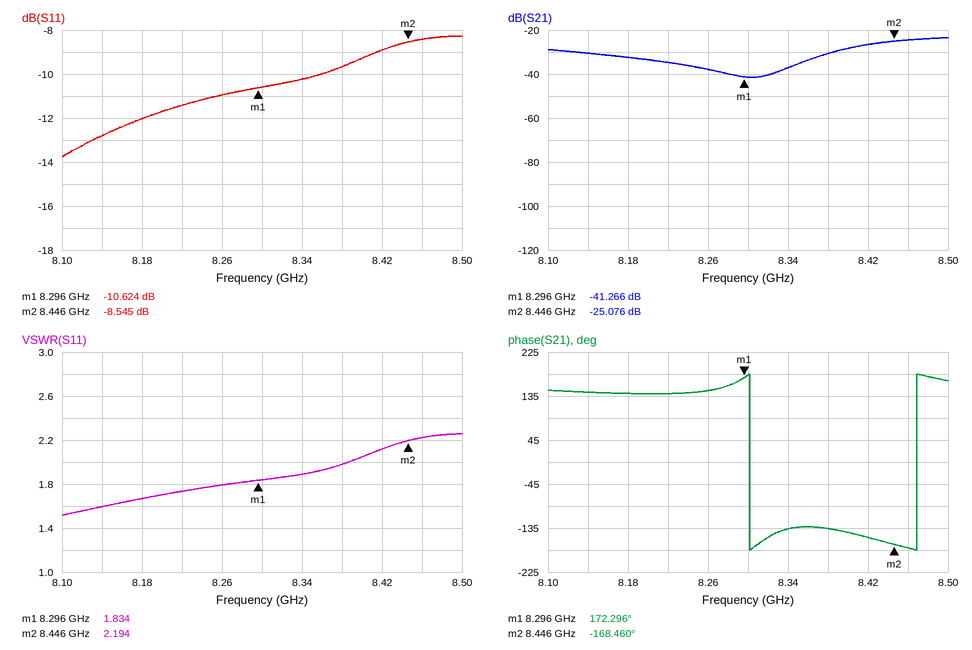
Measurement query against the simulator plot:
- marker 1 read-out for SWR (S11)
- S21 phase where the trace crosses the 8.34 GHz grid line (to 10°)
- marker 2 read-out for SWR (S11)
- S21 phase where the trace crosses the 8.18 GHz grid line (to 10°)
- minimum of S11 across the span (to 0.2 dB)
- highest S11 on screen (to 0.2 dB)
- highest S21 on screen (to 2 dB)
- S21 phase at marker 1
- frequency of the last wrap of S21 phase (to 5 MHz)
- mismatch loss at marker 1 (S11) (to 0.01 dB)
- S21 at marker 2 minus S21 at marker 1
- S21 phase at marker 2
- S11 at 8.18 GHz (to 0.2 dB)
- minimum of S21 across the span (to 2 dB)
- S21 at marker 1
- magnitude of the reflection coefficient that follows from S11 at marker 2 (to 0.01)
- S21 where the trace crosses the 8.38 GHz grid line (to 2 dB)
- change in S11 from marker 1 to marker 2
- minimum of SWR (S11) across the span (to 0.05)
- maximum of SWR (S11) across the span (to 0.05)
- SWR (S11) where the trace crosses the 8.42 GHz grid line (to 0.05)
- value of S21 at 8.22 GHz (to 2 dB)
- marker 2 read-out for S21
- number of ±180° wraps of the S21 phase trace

1.834
-140°
2.194
140°
-13.8 dB
-8.2 dB
-24 dB
172.296°
8.470 GHz
0.39 dB
16.190 dB
-168.460°
-12.0 dB
-42 dB
-41.266 dB
0.37
-30 dB
2.079 dB
1.50
2.25
2.10
-34 dB
-25.076 dB
2
